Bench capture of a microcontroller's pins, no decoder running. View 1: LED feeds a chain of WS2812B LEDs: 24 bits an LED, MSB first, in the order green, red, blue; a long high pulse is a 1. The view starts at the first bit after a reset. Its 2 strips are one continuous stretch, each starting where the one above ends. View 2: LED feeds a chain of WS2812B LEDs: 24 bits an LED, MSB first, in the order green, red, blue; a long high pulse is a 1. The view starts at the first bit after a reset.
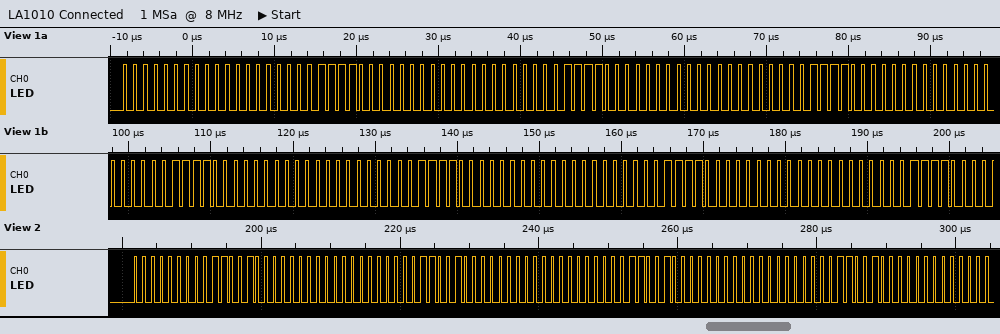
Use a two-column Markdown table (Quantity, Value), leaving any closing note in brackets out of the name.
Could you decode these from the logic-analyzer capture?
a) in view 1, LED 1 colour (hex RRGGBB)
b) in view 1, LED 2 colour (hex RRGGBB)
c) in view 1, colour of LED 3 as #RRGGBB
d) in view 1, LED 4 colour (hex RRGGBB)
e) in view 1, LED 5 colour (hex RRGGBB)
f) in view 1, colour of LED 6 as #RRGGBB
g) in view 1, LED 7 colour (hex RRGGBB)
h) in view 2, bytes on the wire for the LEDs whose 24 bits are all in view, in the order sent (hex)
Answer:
| Quantity | Value |
|---|---|
| in view 1, LED 1 colour | #00001E |
| in view 1, LED 2 colour | #00001E |
| in view 1, colour of LED 3 as #RRGGBB | #00001E |
| in view 1, LED 4 colour | #00001E |
| in view 1, LED 5 colour | #00001E |
| in view 1, colour of LED 6 as #RRGGBB | #00001E |
| in view 1, LED 7 colour | #00001E |
| in view 2, bytes on the wire for the LEDs whose 24 bits are all in view, in the order sent | 00 64 00 00 64 00 00 64 00 00 64 00 |
